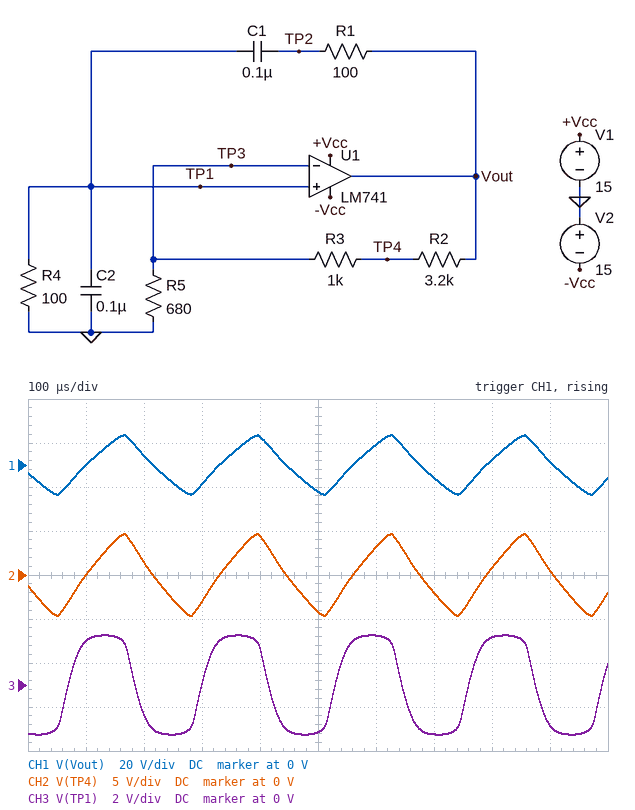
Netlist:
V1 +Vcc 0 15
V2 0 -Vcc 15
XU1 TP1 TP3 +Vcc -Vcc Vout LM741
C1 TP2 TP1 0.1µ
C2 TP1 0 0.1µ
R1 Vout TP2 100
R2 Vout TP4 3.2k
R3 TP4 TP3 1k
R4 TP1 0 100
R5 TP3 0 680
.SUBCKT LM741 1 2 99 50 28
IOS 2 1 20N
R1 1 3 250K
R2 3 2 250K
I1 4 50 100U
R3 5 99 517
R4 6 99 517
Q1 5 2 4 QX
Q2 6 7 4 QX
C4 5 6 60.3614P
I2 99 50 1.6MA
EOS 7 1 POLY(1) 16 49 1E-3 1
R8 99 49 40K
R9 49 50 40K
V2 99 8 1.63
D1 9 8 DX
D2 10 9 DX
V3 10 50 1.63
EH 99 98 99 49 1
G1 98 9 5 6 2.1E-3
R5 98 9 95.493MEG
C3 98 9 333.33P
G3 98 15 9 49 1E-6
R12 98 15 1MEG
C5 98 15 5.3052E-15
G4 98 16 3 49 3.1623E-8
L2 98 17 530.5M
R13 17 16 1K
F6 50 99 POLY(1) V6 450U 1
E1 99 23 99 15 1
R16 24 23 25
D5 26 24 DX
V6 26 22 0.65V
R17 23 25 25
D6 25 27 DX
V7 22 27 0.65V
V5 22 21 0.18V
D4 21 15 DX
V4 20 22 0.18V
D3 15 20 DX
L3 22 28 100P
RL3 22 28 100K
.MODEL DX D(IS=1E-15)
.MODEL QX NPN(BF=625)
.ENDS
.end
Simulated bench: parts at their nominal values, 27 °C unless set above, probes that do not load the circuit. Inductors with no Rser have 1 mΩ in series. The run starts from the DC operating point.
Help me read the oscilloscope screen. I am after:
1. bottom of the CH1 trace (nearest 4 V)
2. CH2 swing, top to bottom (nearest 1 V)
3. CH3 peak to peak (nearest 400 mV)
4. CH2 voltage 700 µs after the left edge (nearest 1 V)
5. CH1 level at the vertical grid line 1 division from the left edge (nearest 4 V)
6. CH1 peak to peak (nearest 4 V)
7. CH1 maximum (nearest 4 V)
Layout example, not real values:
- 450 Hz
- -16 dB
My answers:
- -12 V
- 9 V
- 4.4 V
- -2 V
- 0 V
- 28 V
- 12 V
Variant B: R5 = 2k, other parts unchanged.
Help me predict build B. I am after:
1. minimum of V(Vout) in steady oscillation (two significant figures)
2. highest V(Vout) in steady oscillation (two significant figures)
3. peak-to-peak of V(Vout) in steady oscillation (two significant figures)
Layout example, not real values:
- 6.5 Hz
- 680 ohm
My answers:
- -5.1 V
- 5.1 V
- 10 V
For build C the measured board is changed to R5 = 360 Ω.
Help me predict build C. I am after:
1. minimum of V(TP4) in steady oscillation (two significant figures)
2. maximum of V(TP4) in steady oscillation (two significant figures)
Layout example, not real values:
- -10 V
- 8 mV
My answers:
- -4.1 V
- 4.1 V
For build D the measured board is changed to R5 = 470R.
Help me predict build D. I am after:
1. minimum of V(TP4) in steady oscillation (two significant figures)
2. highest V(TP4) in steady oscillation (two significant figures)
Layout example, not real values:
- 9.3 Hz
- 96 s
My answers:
- -4.3 V
- 4.3 V
